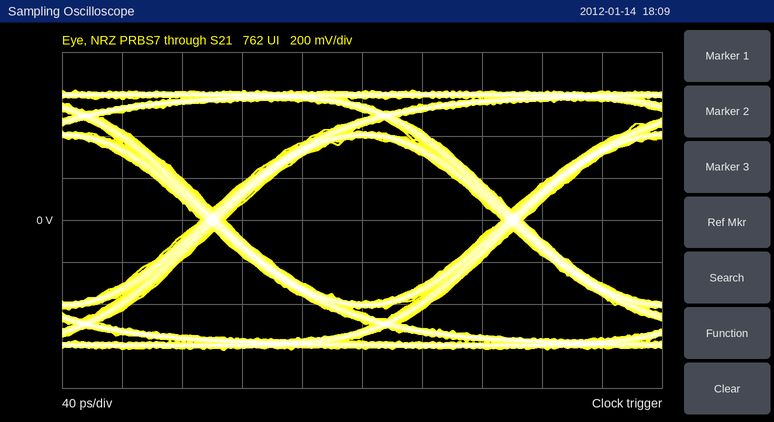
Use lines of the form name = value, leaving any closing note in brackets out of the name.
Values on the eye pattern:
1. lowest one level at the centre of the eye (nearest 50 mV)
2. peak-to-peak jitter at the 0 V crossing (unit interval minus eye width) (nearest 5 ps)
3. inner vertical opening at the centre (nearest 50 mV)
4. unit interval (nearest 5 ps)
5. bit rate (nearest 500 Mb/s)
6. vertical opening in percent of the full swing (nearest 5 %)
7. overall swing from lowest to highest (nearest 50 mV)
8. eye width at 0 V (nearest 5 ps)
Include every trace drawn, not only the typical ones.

lowest one level at the centre of the eye = 400 mV
peak-to-peak jitter at the 0 V crossing (unit interval minus eye width) = 15 ps
inner vertical opening at the centre = 800 mV
unit interval = 200 ps
bit rate = 5.0 Gb/s
vertical opening in percent of the full swing = 65 %
overall swing from lowest to highest = 1.25 V
eye width at 0 V = 185 ps
